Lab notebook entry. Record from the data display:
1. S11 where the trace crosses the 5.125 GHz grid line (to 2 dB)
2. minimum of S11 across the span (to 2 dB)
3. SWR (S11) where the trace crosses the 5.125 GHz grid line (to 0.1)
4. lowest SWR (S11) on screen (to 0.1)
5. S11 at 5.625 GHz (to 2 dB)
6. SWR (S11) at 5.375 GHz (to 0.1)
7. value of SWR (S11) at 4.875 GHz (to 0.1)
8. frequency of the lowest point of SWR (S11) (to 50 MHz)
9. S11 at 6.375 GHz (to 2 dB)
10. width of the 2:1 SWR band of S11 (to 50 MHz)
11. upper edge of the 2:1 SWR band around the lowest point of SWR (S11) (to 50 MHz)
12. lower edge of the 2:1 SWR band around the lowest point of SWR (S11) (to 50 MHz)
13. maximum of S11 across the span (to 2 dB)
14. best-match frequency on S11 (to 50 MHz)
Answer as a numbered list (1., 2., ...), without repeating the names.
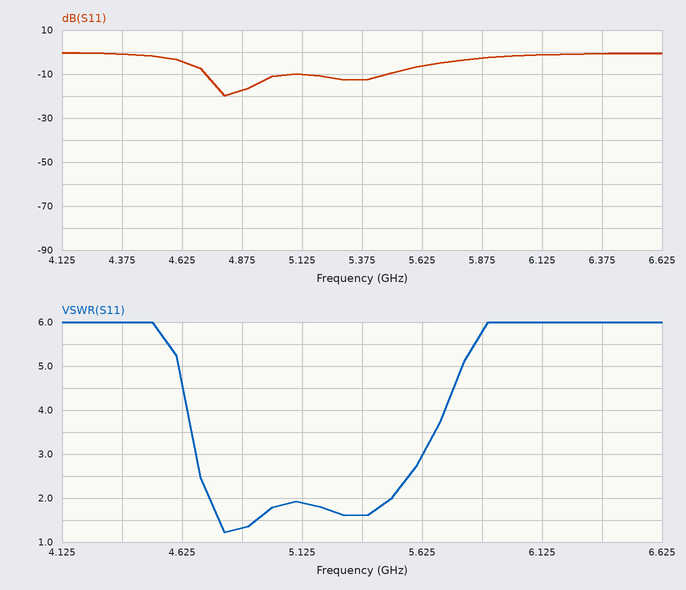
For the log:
1. -10 dB
2. -20 dB
3. 1.9
4. 1.2
5. -6 dB
6. 1.6
7. 1.3
8. 4.80 GHz
9. 0 dB
10. 750 MHz
11. 5.50 GHz
12. 4.75 GHz
13. 0 dB
14. 4.80 GHz
